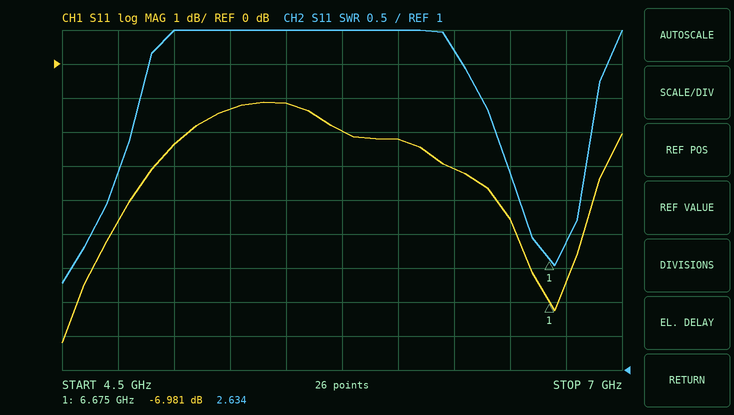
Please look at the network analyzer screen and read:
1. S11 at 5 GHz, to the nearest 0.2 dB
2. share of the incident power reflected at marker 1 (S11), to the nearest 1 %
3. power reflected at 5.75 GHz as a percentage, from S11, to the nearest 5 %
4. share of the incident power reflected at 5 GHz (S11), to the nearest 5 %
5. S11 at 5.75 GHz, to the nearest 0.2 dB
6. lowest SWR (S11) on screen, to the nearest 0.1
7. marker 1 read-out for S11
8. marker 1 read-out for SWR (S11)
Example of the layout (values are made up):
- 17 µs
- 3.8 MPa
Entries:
- -2.4 dB
- 20 %
- 65 %
- 60 %
- -2.0 dB
- 2.3
- -6.981 dB
- 2.634
